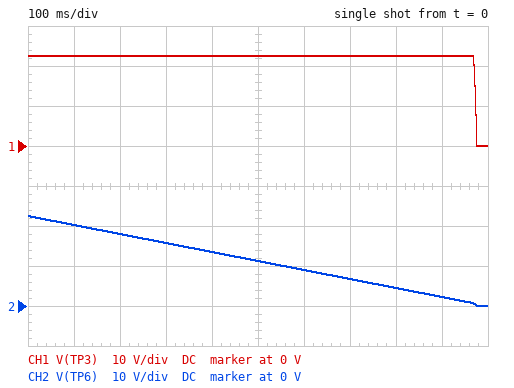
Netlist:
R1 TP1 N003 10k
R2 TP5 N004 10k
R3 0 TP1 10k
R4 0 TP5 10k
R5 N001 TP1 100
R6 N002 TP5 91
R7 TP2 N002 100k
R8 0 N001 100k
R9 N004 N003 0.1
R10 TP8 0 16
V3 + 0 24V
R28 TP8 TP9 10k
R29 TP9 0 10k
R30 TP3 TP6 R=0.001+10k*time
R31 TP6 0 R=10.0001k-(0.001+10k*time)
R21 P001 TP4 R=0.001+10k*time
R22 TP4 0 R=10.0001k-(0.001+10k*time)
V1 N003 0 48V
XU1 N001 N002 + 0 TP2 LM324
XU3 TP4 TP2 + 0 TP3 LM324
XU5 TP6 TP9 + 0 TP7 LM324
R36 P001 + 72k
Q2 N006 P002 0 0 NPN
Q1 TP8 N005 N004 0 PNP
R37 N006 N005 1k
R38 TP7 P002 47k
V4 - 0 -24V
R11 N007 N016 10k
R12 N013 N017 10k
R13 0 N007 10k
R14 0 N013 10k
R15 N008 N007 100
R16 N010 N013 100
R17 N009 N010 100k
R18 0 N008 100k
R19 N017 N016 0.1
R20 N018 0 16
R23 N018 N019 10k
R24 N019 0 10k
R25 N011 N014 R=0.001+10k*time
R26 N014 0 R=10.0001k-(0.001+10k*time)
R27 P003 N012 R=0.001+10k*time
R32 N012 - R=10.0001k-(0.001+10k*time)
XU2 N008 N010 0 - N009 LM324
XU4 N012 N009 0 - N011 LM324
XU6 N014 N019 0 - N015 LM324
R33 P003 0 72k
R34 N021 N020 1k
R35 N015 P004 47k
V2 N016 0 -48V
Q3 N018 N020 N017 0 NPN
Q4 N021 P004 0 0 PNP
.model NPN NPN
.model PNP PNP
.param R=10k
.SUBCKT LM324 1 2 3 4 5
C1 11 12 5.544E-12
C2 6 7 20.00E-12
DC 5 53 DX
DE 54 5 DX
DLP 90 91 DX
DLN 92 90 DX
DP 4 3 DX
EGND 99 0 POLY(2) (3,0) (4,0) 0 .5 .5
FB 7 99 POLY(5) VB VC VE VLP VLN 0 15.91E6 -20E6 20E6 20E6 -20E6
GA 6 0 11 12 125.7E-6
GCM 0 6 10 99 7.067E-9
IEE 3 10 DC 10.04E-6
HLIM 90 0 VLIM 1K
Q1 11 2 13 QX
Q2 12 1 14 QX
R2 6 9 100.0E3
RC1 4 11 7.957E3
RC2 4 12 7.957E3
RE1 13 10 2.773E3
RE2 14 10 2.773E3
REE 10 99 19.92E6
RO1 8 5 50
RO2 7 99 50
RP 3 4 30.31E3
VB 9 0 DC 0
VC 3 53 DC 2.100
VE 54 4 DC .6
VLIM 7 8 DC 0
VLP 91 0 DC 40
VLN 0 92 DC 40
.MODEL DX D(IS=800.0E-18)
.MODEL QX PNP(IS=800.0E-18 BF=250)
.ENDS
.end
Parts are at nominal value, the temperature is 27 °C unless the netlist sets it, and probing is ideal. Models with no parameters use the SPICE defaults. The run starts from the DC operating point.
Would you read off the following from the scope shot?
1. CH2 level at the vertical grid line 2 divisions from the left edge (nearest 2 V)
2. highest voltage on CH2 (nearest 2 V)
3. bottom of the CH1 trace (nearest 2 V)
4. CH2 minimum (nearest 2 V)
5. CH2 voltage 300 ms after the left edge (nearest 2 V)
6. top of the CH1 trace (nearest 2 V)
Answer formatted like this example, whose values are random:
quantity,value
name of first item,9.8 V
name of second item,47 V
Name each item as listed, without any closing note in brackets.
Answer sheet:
quantity,value
CH2 level at the vertical grid line 2 divisions from the left edge,18 V
highest voltage on CH2,22 V
bottom of the CH1 trace,0 V
CH2 minimum,0 V
CH2 voltage 300 ms after the left edge,16 V
top of the CH1 trace,22 V
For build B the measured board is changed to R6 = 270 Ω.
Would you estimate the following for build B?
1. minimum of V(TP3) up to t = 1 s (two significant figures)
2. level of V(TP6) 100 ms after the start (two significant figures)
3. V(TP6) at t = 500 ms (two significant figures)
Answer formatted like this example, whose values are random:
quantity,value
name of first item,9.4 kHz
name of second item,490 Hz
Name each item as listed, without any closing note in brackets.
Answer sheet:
quantity,value
minimum of V(TP3) up to t = 1 s,3.4 mV
level of V(TP6) 100 ms after the start,16 V
V(TP6) at t = 500 ms,6.1 V
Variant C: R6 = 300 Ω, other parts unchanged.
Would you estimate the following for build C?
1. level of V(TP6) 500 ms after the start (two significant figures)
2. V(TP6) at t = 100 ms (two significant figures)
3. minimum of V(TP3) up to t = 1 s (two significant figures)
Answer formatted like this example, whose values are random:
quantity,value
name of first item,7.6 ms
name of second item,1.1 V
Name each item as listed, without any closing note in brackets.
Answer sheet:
quantity,value
level of V(TP6) 500 ms after the start,5.1 V
V(TP6) at t = 100 ms,15 V
minimum of V(TP3) up to t = 1 s,3.4 mV
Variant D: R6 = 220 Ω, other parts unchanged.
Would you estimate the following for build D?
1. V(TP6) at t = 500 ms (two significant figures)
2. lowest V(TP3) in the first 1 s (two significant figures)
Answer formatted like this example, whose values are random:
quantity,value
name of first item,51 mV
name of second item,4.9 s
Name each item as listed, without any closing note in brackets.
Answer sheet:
quantity,value
V(TP6) at t = 500 ms,7.8 V
lowest V(TP3) in the first 1 s,3.4 mV
